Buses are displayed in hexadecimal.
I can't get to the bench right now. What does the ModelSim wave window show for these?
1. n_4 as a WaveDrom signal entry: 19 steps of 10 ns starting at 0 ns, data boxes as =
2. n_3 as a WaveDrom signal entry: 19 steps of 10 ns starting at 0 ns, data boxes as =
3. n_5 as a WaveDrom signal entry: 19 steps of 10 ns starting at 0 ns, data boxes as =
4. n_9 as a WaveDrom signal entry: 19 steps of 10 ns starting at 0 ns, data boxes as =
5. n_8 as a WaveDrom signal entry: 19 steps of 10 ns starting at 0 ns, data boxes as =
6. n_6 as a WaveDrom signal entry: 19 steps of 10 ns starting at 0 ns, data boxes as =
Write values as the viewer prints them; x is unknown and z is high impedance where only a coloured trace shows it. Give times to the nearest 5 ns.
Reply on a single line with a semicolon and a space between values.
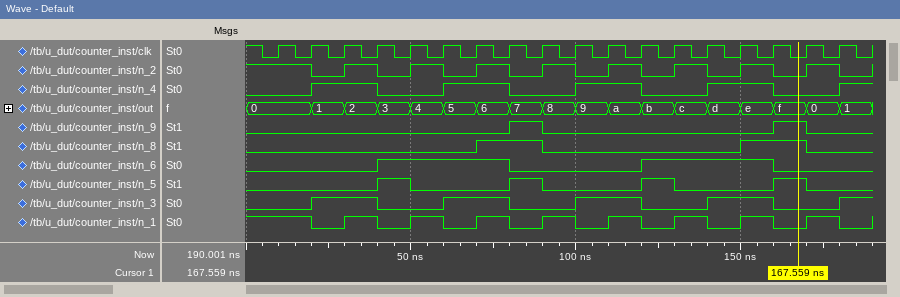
{name: 'n_4', wave: '0.1.0.1.0.1.0.1.0.1'}; {name: 'n_3', wave: '0.1.0.1.0.1.0.1.0.1'}; {name: 'n_5', wave: '0...10..10..10..10.'}; {name: 'n_9', wave: '0.......10......10.'}; {name: 'n_8', wave: '0......1.0.....1.0.'}; {name: 'n_6', wave: '0...1...0...1...0..'}
